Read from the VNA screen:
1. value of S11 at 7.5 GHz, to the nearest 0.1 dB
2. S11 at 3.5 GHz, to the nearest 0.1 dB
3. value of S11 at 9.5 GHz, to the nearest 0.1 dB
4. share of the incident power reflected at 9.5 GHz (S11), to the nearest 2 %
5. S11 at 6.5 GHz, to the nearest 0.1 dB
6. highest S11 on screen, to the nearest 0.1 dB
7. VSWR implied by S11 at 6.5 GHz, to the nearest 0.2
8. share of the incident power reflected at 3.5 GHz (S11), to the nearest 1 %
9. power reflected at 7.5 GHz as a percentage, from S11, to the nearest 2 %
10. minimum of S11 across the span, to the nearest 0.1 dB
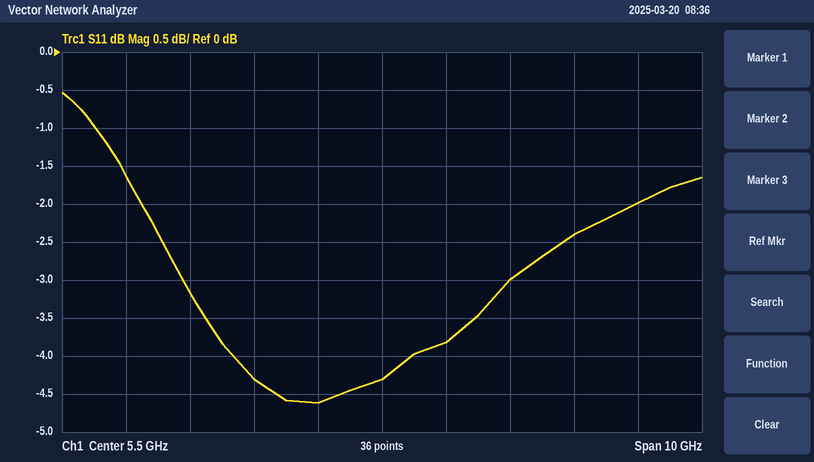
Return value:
-3.0 dB
-4.3 dB
-2.0 dB
64 %
-3.8 dB
-0.5 dB
4.6
37 %
50 %
-4.6 dB
